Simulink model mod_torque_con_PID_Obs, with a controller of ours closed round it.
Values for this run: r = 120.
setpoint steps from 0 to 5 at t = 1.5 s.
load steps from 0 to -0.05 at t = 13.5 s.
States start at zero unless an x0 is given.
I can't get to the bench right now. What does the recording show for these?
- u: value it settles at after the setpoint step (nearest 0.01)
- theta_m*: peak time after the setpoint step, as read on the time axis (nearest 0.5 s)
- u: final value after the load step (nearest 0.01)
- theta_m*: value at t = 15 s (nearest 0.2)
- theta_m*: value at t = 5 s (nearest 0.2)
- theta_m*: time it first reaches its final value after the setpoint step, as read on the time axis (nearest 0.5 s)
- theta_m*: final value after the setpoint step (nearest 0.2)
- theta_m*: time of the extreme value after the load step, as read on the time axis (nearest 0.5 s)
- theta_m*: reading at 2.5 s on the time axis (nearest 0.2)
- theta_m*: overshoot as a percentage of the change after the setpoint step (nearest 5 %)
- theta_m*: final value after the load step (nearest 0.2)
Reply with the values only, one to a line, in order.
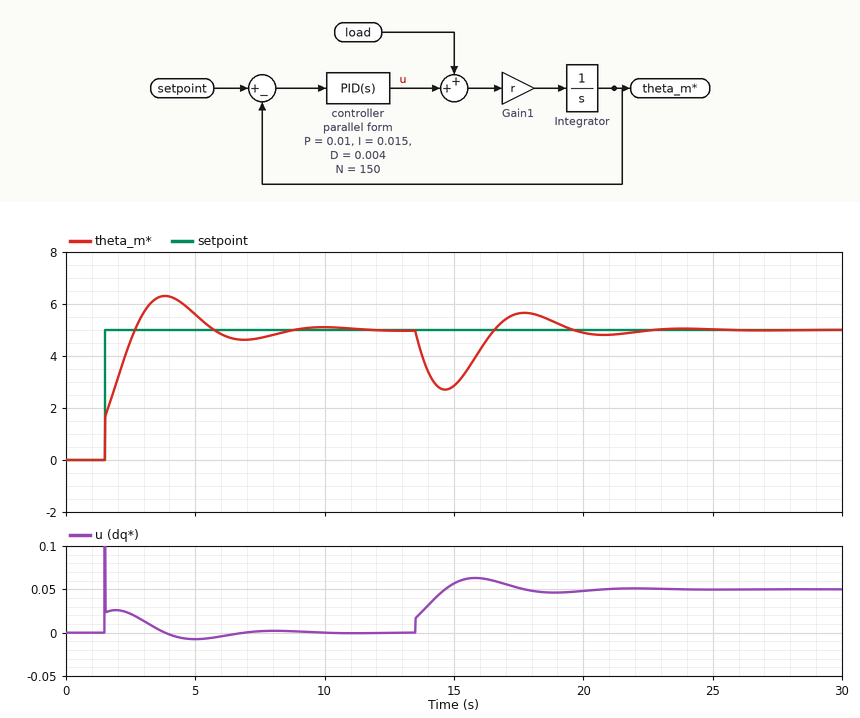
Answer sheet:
0.00
4.0 s
0.05
2.8
5.6
2.5 s
5.0
14.5 s
4.6
25 %
5.0
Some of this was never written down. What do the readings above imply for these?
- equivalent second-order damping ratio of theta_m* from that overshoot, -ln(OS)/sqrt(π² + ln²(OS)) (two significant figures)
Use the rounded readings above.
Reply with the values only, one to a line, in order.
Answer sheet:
0.40
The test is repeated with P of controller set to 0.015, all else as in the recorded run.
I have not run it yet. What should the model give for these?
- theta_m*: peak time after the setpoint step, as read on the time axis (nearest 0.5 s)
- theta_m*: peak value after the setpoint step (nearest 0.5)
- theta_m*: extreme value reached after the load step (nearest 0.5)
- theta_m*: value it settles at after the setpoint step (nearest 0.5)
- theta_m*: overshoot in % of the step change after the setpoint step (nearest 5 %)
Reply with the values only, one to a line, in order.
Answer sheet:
3.5 s
6.0
3.0
5.0
20 %
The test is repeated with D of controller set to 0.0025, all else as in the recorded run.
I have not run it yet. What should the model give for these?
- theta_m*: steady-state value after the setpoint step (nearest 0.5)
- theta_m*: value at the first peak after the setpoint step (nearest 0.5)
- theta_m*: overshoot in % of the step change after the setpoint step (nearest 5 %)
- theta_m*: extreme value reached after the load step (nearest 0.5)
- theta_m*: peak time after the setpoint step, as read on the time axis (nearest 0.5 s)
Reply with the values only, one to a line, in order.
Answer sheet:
5.0
6.5
30 %
2.5
3.5 s
